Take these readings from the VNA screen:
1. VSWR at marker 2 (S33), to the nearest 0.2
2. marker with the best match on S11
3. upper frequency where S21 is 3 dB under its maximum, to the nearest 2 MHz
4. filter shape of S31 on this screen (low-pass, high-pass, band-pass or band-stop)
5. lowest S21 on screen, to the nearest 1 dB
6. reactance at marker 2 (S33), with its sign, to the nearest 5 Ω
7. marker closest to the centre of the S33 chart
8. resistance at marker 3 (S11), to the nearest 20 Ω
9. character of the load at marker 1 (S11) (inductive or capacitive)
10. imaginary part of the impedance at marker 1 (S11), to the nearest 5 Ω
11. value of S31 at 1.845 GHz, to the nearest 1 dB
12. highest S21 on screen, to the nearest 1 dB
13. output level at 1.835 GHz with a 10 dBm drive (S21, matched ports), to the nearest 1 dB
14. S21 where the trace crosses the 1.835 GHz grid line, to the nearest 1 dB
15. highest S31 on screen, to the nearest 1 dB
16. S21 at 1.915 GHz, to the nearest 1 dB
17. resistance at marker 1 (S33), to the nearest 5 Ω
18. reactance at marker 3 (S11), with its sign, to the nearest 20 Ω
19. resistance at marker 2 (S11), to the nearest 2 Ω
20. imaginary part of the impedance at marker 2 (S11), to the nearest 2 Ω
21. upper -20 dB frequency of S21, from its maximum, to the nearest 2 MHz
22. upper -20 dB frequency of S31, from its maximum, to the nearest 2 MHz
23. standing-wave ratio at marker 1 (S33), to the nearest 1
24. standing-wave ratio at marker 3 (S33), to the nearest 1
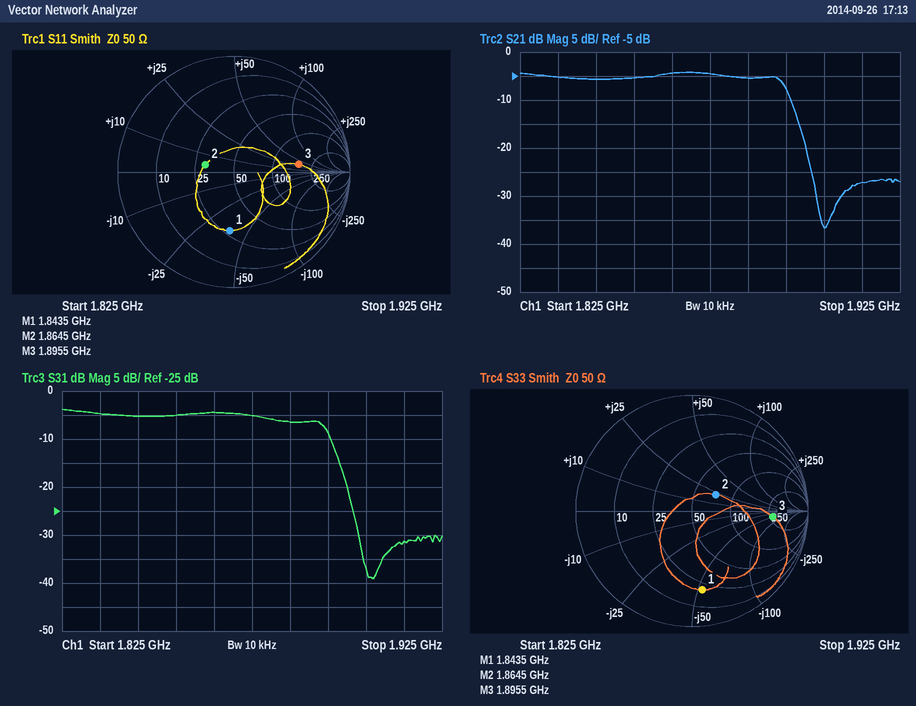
1.6
marker 2
1.894 GHz
low-pass
-37 dB
+20 Ω
marker 2
180 Ω
capacitive
-40 Ω
-5 dB
-4 dB
5 dBm
-5 dB
-4 dB
-27 dB
20 Ω
+40 Ω
30 Ω
+4 Ω
1.902 GHz
1.902 GHz
5
6
